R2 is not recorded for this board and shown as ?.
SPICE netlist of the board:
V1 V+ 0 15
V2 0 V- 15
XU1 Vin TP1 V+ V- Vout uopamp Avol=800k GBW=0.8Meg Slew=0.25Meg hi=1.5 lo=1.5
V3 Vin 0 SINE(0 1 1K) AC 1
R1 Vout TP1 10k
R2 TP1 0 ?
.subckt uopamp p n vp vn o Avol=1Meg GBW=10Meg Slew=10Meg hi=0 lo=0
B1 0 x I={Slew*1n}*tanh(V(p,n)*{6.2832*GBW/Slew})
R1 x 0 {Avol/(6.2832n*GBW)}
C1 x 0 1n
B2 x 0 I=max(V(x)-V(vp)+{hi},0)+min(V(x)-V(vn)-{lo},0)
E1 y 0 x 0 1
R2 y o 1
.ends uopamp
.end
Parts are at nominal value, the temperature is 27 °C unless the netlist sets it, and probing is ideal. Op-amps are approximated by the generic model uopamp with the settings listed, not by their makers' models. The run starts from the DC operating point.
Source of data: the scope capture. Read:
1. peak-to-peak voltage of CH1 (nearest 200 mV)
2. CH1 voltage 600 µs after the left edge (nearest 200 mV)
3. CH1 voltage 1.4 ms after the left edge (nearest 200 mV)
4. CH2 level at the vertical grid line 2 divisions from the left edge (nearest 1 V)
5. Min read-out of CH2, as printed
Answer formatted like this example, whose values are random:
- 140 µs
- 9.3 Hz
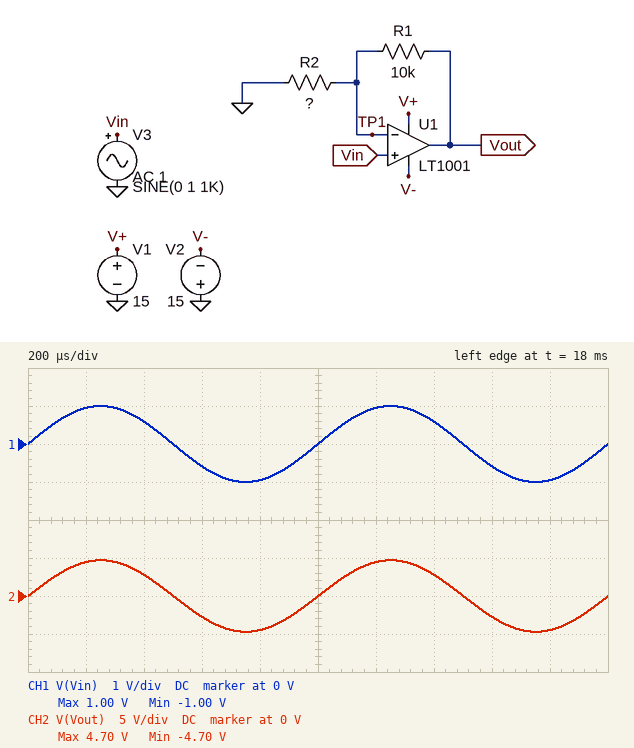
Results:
- 2.0 V
- -600 mV
- 600 mV
- 3 V
- -4.70 V
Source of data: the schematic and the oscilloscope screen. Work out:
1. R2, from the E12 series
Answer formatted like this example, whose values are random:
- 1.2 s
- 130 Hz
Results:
- 2.7 kΩ
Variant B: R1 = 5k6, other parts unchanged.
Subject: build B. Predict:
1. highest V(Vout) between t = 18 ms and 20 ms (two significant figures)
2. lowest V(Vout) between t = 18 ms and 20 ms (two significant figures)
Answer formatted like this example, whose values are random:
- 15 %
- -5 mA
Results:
- 3.1 V
- -3.1 V
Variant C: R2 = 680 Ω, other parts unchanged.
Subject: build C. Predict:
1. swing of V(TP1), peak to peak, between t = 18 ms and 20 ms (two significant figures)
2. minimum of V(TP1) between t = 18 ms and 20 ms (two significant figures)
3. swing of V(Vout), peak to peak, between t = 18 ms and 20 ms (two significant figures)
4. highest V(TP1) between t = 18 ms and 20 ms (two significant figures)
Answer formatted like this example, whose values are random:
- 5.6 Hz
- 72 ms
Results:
- 1.7 V
- -860 mV
- 27 V
- 860 mV
